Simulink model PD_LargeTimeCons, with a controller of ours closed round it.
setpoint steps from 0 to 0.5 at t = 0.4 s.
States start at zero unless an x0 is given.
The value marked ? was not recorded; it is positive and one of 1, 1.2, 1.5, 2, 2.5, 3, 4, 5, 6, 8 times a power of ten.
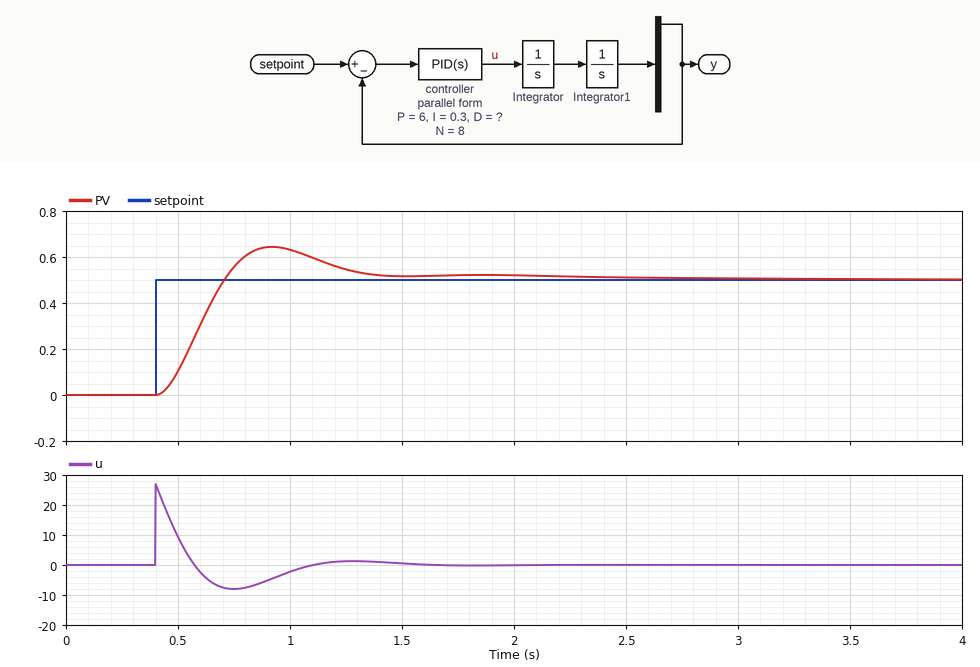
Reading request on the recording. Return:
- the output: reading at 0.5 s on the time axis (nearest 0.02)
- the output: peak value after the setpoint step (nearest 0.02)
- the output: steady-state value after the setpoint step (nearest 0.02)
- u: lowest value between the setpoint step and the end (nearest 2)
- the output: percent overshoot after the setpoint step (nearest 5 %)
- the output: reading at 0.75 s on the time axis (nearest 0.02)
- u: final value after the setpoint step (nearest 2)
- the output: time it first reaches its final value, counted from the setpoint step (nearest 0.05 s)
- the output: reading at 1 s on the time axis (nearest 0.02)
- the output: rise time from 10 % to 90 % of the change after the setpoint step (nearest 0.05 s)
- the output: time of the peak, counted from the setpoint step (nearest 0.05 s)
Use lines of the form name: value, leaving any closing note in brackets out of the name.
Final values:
the output: reading at 0.5 s on the time axis: 0.10
the output: peak value after the setpoint step: 0.64
the output: steady-state value after the setpoint step: 0.50
u: lowest value between the setpoint step and the end: -8
the output: percent overshoot after the setpoint step: 30 %
the output: reading at 0.75 s on the time axis: 0.56
u: final value after the setpoint step: 0
the output: time it first reaches its final value, counted from the setpoint step: 0.30 s
the output: reading at 1 s on the time axis: 0.64
the output: rise time from 10 % to 90 % of the change after the setpoint step: 0.20 s
the output: time of the peak, counted from the setpoint step: 0.50 s
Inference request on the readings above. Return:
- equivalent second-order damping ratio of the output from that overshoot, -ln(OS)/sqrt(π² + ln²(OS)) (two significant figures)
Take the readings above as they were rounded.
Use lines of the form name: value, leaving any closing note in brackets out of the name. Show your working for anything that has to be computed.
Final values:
equivalent second-order damping ratio of the output from that overshoot, -ln(OS)/sqrt(π² + ln²(OS)): ln(0.3) = -1.204; 1.204 / sqrt(9.870 + 1.450) = 0.36
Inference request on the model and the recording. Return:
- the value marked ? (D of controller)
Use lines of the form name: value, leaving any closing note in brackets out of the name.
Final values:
the value marked ?: 6
